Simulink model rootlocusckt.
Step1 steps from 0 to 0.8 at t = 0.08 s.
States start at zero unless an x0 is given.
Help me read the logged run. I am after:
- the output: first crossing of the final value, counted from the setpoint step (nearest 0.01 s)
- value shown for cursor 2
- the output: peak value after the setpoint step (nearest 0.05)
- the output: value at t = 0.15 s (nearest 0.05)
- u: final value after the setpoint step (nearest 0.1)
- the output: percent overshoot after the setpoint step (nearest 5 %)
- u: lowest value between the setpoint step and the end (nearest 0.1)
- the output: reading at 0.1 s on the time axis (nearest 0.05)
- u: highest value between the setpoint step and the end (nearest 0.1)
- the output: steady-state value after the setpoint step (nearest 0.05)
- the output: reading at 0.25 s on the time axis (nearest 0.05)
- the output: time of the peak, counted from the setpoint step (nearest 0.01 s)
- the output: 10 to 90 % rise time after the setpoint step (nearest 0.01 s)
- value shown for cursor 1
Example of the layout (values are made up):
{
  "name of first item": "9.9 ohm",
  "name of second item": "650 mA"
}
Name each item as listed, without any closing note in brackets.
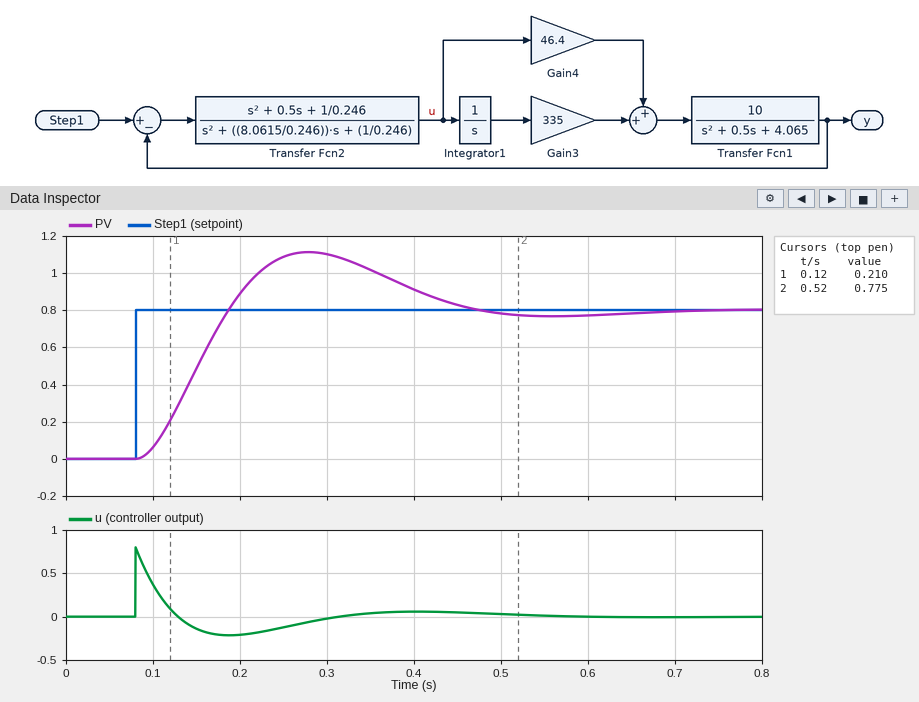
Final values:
{
  "the output: first crossing of the final value, counted from the setpoint step": "0.11 s",
  "value shown for cursor 2": "0.775",
  "the output: peak value after the setpoint step": "1.10",
  "the output: value at t = 0.15 s": "0.50",
  "u: final value after the setpoint step": "0.0",
  "the output: percent overshoot after the setpoint step": "40 %",
  "u: lowest value between the setpoint step and the end": "-0.2",
  "the output: reading at 0.1 s on the time axis": "0.05",
  "u: highest value between the setpoint step and the end": "0.8",
  "the output: steady-state value after the setpoint step": "0.80",
  "the output: reading at 0.25 s on the time axis": "1.10",
  "the output: time of the peak, counted from the setpoint step": "0.20 s",
  "the output: 10 to 90 % rise time after the setpoint step": "0.07 s",
  "value shown for cursor 1": "0.210"
}
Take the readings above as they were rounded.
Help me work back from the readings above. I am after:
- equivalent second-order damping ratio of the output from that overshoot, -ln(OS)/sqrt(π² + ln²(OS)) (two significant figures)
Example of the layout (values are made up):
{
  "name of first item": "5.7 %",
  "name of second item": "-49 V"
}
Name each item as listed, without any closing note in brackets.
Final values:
{
  "equivalent second-order damping ratio of the output from that overshoot, -ln(OS)/sqrt(π² + ln²(OS))": "0.28"
}
